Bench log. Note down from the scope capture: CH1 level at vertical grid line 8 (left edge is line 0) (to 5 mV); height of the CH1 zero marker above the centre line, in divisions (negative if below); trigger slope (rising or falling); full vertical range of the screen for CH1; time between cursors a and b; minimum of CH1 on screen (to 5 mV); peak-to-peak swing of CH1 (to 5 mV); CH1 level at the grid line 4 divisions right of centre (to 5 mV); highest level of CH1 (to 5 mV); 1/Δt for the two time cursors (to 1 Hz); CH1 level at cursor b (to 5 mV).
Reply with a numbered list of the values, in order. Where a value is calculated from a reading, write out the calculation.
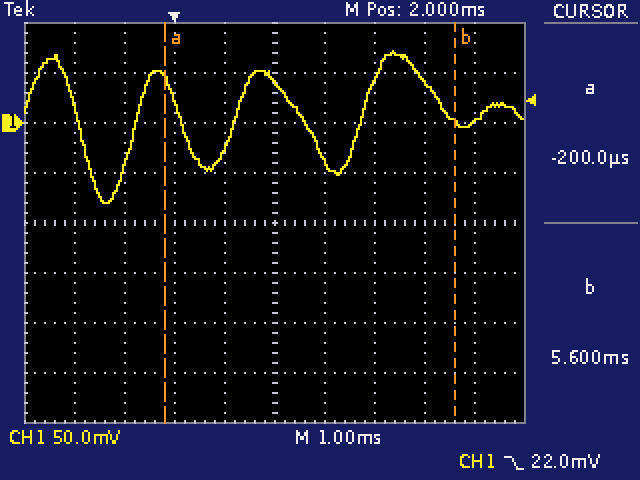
1. 40 mV
2. +2.0 div
3. falling
4. 400 mV
5. 5.6 ms − (-200 µs) = 5.8 ms
6. -80 mV
7. 70 mV − (-80 mV) = 150 mV
8. 0 mV
9. 70 mV
10. 1 / 5.8 ms ≈ 172 Hz
11. 0 mV
